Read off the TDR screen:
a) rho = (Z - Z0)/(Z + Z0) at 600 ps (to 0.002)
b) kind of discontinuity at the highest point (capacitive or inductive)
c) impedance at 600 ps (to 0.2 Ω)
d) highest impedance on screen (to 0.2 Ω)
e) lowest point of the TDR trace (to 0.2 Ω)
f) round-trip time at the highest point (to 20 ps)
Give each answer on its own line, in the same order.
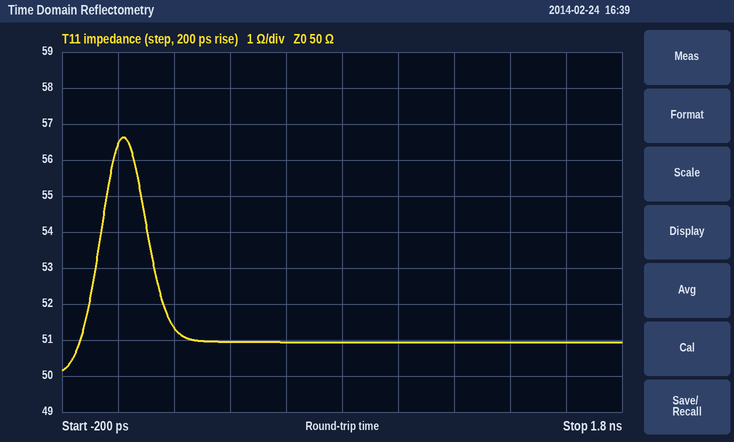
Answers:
+0.010
inductive
51.0 Ω
56.6 Ω
50.2 Ω
20 ps
